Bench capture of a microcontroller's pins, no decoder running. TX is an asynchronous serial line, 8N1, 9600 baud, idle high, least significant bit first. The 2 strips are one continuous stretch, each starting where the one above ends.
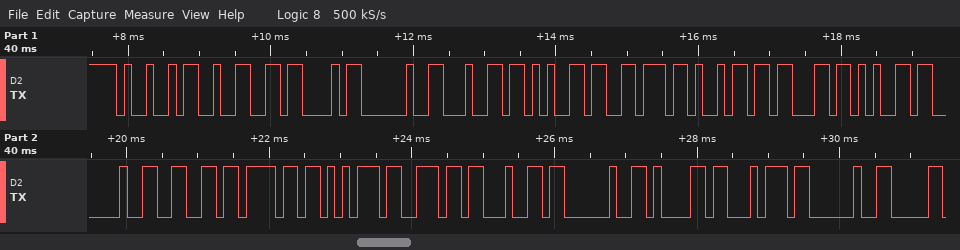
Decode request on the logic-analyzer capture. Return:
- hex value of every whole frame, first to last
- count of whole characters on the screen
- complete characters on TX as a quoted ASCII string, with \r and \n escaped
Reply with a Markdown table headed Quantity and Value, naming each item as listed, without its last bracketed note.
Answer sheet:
| Quantity | Value |
|---|---|
| hex value of every whole frame, first to last | 49 32 43 20 64 65 76 69 63 65 20 66 6F 75 6E 64 20 61 74 20 |
| count of whole characters on the screen | 20 |
| complete characters on TX as a quoted ASCII string, with \r and \n escaped | "I2C device found at " |
